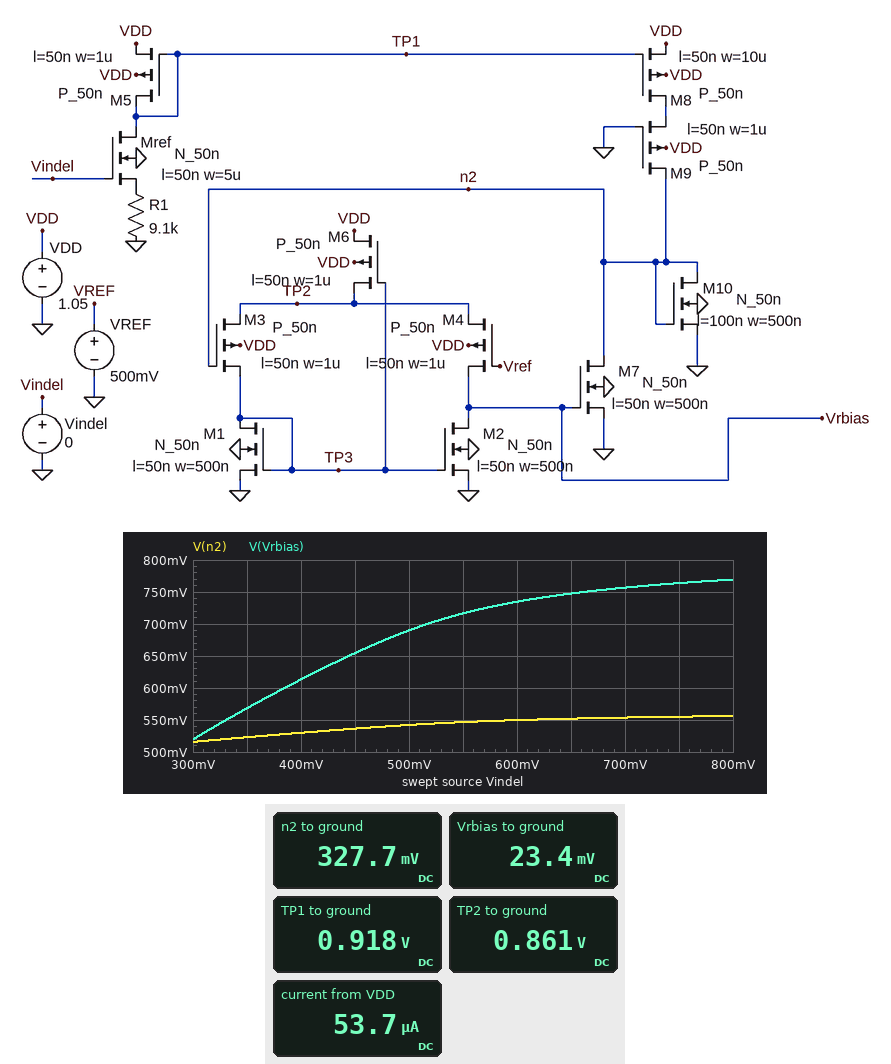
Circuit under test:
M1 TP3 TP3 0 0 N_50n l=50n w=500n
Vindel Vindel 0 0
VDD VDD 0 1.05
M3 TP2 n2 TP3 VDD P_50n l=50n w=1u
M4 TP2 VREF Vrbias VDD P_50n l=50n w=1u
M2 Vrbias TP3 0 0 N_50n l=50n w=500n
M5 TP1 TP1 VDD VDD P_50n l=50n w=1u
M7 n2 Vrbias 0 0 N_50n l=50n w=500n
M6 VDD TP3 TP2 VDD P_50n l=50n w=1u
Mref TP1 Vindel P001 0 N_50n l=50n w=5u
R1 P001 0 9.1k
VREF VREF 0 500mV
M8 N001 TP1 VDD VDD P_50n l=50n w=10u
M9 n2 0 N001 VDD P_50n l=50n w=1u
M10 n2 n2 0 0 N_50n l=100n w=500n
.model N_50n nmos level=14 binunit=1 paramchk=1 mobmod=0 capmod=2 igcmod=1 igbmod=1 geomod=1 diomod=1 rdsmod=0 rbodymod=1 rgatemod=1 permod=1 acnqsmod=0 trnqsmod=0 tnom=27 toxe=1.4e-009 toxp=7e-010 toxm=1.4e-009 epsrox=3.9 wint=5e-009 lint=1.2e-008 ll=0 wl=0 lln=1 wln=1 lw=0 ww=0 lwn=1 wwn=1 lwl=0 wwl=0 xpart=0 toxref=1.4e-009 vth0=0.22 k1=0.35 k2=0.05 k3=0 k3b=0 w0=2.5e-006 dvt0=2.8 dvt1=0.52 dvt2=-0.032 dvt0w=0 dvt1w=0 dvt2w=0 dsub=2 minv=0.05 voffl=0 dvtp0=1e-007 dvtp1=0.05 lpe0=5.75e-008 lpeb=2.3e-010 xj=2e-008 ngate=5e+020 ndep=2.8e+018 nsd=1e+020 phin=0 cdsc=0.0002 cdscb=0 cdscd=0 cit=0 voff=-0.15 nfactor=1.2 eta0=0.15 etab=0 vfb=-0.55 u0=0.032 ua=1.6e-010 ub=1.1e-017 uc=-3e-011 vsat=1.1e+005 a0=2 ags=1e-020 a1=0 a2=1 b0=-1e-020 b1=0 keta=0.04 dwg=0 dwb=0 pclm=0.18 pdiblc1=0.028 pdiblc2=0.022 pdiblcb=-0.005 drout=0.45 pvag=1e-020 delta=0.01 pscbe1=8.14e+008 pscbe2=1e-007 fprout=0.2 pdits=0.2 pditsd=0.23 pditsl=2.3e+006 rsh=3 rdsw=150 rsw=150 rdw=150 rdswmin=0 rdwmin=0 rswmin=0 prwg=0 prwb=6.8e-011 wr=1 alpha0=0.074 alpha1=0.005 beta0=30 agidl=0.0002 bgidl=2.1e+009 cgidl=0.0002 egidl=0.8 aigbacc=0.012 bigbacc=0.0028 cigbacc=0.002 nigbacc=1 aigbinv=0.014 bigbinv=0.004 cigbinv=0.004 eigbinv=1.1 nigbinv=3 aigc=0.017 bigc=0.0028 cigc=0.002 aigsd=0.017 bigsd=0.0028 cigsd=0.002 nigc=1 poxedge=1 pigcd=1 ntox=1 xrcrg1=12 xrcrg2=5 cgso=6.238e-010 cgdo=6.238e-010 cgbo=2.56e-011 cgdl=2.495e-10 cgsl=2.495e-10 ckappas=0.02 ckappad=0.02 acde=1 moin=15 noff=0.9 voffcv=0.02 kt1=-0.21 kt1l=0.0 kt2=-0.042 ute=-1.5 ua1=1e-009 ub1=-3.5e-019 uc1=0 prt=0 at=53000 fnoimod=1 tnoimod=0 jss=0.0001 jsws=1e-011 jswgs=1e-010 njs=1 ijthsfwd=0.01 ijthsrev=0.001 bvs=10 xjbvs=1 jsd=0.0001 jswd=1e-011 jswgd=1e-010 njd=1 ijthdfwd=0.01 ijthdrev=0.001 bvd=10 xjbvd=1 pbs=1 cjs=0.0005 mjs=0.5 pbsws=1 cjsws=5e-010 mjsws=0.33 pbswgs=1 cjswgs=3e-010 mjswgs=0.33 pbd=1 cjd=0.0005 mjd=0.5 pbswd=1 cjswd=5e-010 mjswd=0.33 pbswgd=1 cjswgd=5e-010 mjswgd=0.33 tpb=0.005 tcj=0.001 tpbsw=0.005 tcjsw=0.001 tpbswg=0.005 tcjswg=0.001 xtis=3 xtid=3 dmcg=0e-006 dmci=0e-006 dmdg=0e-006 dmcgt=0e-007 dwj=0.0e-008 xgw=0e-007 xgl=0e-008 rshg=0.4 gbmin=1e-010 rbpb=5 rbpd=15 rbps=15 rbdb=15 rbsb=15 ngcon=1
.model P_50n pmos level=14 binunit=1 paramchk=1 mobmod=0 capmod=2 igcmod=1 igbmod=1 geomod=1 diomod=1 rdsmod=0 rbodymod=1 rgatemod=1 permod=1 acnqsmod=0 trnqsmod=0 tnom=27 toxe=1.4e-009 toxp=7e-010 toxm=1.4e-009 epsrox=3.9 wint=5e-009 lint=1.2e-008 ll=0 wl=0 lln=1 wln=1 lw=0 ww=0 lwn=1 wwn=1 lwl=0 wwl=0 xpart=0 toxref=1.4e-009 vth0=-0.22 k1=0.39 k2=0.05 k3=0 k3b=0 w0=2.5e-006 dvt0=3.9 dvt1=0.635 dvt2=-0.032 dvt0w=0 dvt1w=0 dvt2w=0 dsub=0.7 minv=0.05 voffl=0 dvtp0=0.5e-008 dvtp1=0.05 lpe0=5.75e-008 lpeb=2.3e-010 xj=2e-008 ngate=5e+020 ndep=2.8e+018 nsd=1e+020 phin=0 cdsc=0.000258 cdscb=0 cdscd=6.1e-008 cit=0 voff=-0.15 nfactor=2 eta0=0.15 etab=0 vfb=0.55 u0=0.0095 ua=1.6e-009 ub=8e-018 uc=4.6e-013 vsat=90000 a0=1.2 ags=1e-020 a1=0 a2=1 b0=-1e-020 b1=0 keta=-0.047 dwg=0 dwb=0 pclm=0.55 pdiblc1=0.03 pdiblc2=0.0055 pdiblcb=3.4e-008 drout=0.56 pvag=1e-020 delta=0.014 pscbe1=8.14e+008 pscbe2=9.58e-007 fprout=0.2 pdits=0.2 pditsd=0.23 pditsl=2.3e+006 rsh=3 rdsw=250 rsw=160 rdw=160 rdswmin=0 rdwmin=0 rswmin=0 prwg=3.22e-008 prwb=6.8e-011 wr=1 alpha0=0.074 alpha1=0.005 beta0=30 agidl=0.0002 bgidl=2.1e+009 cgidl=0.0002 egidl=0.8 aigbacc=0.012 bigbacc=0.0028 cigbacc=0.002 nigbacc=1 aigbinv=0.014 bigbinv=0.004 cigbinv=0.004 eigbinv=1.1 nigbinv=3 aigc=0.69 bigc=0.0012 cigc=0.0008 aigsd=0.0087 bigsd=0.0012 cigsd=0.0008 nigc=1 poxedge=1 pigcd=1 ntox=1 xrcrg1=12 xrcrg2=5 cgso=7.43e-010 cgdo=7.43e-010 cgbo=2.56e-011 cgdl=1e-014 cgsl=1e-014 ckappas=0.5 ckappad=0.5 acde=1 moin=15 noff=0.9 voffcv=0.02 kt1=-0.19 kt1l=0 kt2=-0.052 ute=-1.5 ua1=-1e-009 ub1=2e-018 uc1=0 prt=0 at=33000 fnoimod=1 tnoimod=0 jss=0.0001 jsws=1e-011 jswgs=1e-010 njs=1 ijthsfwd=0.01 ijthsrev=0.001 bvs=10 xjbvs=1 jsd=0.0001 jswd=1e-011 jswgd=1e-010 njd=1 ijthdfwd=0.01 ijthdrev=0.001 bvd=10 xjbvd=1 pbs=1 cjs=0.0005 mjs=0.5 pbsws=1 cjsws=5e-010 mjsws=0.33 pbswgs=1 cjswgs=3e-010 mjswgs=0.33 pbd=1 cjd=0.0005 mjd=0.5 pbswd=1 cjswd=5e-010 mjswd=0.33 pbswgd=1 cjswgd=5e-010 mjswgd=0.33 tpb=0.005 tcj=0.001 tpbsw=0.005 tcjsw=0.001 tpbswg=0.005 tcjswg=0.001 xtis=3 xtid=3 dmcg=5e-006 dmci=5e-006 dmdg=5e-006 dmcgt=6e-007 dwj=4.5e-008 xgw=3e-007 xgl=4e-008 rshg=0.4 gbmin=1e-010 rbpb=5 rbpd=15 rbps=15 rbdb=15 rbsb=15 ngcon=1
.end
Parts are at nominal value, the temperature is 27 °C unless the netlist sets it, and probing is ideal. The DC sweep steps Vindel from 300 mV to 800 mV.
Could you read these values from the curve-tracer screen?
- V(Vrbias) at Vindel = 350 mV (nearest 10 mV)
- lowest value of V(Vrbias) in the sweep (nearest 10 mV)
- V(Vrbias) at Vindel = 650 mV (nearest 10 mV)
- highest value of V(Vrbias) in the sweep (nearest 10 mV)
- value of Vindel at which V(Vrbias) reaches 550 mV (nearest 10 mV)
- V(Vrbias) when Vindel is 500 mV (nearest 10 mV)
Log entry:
570 mV
520 mV
750 mV
770 mV
330 mV
690 mV
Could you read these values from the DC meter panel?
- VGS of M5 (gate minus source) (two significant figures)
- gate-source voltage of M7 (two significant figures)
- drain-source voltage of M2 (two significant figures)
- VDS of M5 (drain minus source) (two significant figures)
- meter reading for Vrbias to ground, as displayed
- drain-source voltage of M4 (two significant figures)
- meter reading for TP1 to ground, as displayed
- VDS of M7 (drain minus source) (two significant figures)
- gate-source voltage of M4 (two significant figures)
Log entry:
-130 mV
23 mV
23 mV
-130 mV
23.4 mV
840 mV
0.918 V
330 mV
480 mV
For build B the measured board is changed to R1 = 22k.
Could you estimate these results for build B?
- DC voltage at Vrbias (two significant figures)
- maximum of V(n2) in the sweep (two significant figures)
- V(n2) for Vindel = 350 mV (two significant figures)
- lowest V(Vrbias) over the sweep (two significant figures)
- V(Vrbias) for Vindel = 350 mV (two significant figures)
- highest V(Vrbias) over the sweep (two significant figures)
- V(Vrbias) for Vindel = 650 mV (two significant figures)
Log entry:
23 mV
540 mV
510 mV
450 mV
480 mV
680 mV
620 mV
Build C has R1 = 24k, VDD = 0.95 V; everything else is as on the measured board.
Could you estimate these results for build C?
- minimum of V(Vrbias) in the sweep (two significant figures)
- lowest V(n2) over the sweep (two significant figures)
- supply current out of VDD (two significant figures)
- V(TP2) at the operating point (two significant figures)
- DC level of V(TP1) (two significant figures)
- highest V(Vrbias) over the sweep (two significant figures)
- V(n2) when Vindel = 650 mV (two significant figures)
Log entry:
420 mV
510 mV
34 µA
800 mV
830 mV
620 mV
530 mV
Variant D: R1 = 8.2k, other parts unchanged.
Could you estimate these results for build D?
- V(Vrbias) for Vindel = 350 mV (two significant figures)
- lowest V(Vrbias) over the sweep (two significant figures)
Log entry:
580 mV
530 mV
